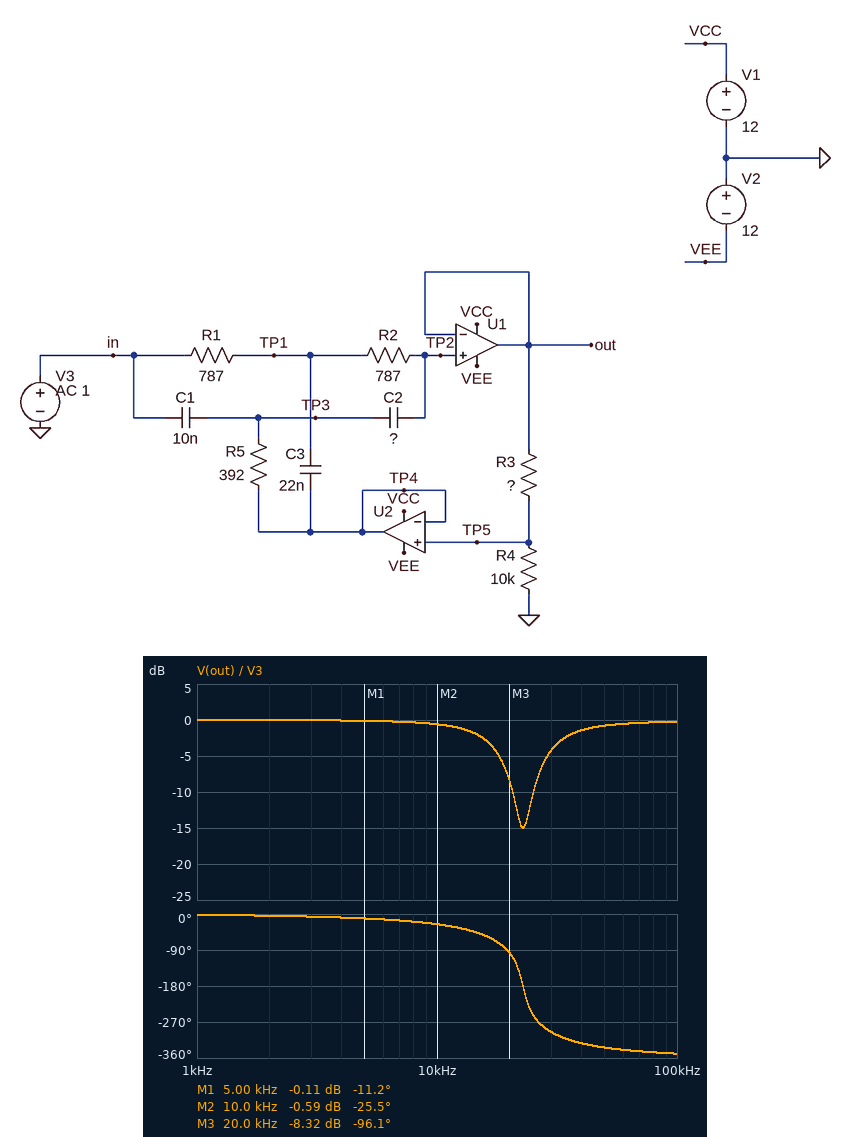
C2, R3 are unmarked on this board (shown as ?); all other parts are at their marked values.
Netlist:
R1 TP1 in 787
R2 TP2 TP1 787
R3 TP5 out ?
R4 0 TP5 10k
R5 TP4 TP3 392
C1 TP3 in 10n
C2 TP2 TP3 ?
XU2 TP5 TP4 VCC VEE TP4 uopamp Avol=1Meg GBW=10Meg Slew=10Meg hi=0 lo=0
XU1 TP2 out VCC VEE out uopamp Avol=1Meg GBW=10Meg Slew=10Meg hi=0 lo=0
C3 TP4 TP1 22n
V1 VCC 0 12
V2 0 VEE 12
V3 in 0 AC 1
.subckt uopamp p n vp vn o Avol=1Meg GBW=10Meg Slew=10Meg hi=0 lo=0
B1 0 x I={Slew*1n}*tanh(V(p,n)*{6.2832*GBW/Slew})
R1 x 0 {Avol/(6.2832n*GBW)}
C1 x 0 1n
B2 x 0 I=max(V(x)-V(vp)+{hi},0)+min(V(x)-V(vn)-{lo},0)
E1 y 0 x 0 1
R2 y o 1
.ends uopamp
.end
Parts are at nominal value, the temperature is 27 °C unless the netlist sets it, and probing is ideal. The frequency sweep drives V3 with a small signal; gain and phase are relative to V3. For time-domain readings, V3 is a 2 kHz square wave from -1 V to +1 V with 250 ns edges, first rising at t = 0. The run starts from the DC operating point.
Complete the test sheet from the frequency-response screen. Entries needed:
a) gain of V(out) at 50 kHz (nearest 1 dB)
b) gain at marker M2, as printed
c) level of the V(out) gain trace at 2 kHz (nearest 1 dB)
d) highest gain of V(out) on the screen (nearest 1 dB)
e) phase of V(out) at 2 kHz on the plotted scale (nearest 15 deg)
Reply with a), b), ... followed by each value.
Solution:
a) -1 dB
b) -0.59 dB
c) 0 dB
d) 0 dB
e) 0 deg
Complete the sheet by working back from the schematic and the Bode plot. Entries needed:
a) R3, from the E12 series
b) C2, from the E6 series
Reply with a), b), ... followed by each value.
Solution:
a) 2.7 kΩ
b) 6.8 nF
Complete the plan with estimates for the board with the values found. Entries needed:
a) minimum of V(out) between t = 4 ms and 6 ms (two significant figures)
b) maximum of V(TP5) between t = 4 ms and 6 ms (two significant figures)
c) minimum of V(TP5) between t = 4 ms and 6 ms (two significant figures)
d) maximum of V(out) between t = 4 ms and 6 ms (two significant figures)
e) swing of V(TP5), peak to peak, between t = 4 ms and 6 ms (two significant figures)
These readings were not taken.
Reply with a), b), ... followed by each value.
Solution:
a) -1.3 V
b) 1.0 V
c) -1.0 V
d) 1.3 V
e) 2.1 V
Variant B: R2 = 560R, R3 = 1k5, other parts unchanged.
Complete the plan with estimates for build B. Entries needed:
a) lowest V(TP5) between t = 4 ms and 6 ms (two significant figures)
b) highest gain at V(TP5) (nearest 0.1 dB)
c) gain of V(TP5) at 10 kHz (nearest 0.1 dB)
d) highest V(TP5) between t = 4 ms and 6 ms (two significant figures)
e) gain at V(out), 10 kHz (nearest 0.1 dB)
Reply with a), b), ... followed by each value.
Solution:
a) -1.2 V
b) -1.2 dB
c) -1.4 dB
d) 1.2 V
e) -0.2 dB
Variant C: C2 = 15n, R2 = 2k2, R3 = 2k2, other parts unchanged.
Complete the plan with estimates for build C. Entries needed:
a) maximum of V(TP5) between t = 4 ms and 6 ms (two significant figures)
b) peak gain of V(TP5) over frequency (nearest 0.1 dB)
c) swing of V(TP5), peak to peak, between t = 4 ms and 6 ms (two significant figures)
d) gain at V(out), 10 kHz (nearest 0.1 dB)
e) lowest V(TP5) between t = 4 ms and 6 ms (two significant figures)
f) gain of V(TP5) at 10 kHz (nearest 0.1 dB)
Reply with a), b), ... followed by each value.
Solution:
a) 1.1 V
b) -1.7 dB
c) 2.2 V
d) -8.1 dB
e) -1.1 V
f) -9.8 dB
